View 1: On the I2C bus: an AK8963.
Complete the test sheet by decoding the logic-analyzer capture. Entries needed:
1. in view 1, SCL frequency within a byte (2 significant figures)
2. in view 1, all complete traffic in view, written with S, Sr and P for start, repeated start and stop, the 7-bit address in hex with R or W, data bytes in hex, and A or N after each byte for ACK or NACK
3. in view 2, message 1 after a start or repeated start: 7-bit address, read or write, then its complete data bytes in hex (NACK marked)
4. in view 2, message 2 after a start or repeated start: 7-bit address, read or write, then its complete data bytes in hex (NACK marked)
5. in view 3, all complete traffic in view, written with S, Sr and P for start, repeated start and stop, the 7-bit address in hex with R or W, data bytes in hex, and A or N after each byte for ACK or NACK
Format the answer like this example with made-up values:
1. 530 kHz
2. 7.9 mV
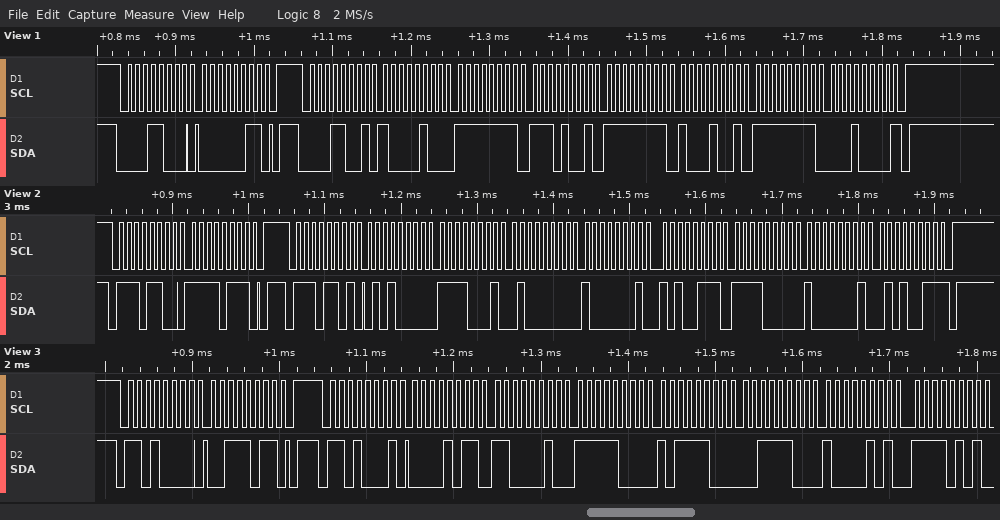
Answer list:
1. 100 kHz
2. S 0CW A 03 A P S 0CR A 84 A FF A E9 A FF A 89 A FF A 10 N P
3. 0x76 write: F7
4. 0x76 read: 50 F1 40 81 A7 F0 81 53 NACK
5. S 68W A 3B A P S 68R A 0B A C2 A F8 A BC A 3C A 85 A F5 A
